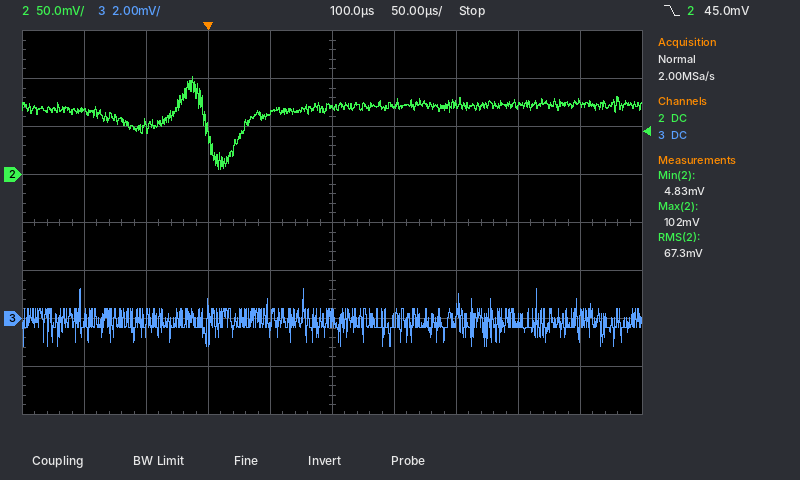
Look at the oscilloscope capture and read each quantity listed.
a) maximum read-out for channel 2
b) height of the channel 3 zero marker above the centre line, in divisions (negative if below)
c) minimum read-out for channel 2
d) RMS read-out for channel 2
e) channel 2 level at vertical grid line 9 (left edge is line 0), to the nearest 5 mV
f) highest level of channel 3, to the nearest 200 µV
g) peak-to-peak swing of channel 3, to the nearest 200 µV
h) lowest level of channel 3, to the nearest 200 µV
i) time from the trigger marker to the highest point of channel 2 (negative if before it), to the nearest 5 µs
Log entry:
102 mV
-2.0 div
4.83 mV
67.3 mV
75 mV
1.2 mV
2.4 mV
-1.2 mV
-15 µs
